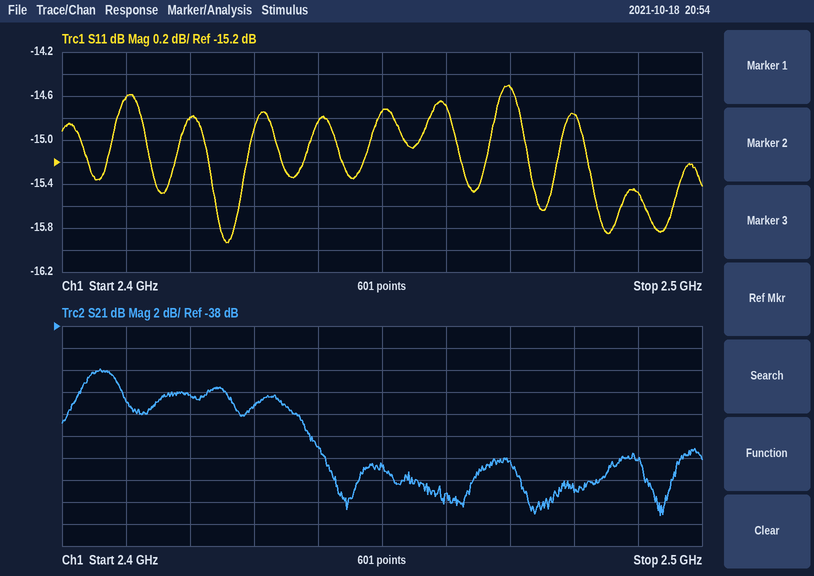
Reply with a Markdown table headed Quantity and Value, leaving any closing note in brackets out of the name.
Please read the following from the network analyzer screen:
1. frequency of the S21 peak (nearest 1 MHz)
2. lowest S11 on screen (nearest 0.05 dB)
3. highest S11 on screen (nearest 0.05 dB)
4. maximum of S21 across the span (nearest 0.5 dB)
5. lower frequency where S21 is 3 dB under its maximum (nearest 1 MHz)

| Quantity | Value |
|---|---|
| frequency of the S21 peak | 2.406 GHz |
| lowest S11 on screen | -15.95 dB |
| highest S11 on screen | -14.50 dB |
| maximum of S21 across the span | -42.0 dB |
| lower frequency where S21 is 3 dB under its maximum | 2.402 GHz |
